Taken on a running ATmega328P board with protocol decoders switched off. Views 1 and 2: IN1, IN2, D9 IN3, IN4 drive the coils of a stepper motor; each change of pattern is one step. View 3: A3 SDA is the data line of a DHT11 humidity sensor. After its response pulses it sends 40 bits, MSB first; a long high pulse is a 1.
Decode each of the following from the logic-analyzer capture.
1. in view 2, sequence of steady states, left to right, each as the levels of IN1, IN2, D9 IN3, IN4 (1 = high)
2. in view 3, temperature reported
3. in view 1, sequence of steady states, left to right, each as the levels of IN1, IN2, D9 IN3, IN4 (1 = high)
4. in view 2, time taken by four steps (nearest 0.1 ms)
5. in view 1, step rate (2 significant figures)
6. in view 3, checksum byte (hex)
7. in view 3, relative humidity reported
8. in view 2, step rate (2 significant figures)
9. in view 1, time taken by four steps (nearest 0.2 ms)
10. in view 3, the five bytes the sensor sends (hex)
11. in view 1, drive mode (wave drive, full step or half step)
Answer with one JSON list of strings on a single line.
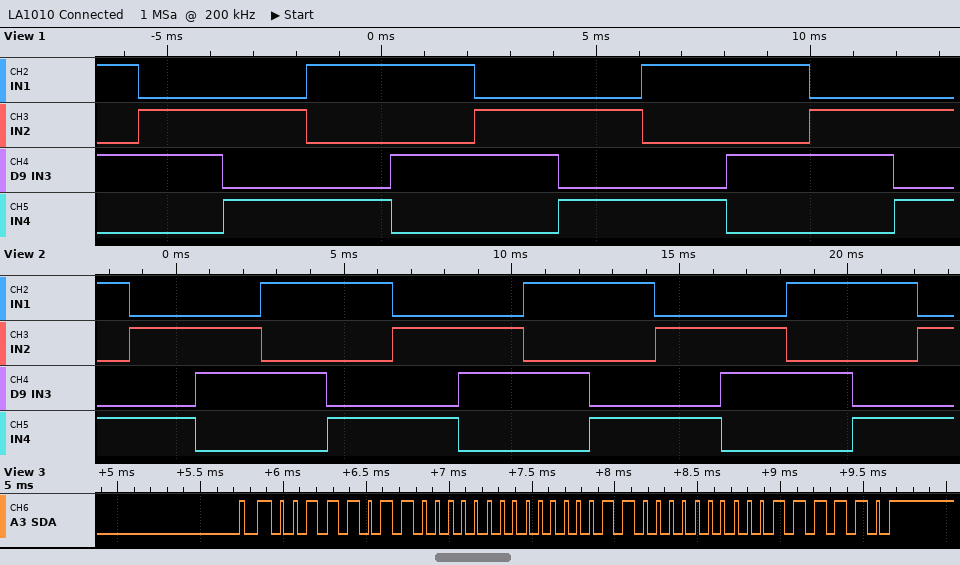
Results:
["1001 0101 0110 1010 1001 0101 0110 1010 1001 0101 0110 1010 1001 0101", "3.0 °C", "1010 0110 0101 1001 1010 0110 0101 1001 1010 0110 0101", "7.8 ms", "510 steps/s", "0x3E", "59 %", "510 steps/s", "7.8 ms", "3B 00 03 00 3E", "full step"]
